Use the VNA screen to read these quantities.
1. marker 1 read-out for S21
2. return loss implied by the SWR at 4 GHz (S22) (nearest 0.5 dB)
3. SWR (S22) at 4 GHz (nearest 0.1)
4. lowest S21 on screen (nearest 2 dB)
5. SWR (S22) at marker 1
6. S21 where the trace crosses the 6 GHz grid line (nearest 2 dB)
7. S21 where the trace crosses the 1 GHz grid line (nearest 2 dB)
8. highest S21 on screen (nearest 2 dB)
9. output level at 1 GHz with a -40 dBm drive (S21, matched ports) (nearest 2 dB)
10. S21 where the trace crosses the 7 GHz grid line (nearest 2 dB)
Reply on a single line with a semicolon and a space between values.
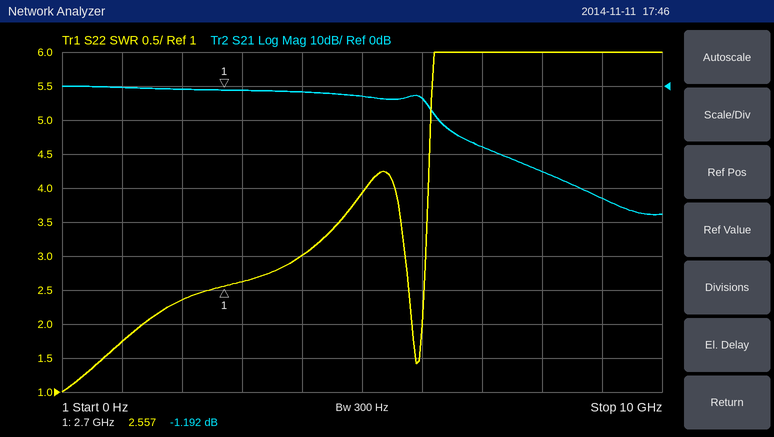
-1.192 dB; 6.0 dB; 3.0; -38 dB; 2.557; -4 dB; 0 dB; 0 dB; -40 dBm; -18 dB
